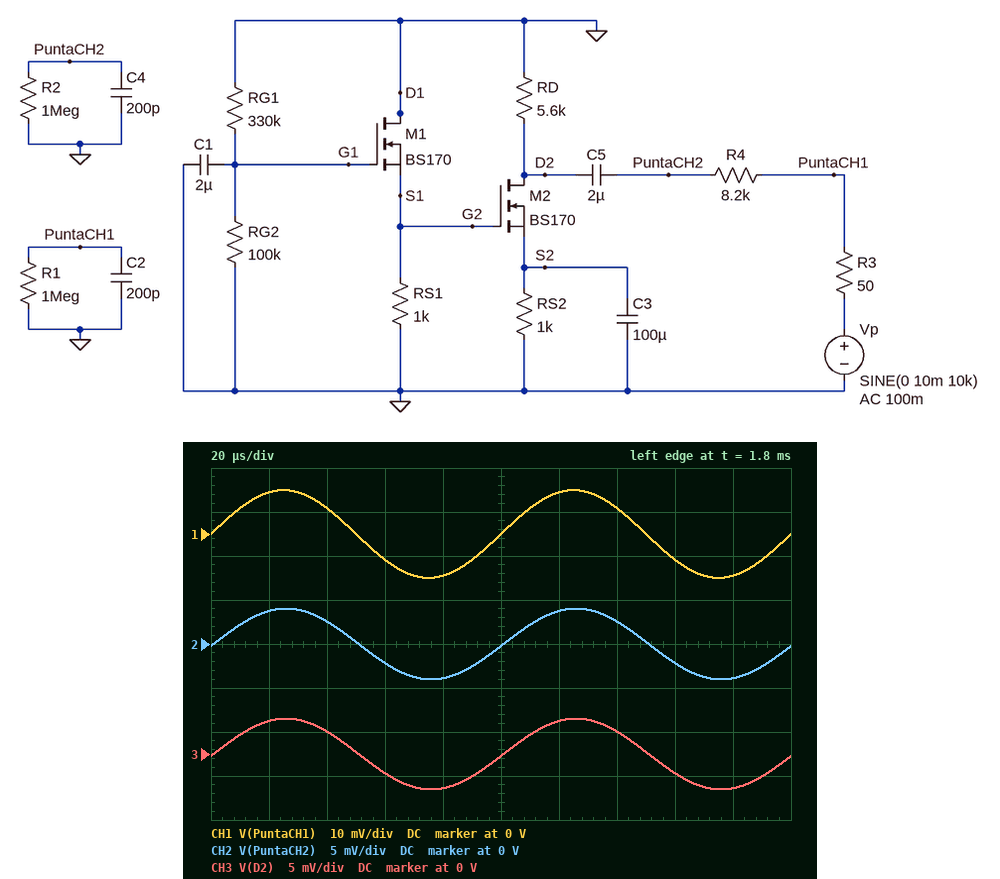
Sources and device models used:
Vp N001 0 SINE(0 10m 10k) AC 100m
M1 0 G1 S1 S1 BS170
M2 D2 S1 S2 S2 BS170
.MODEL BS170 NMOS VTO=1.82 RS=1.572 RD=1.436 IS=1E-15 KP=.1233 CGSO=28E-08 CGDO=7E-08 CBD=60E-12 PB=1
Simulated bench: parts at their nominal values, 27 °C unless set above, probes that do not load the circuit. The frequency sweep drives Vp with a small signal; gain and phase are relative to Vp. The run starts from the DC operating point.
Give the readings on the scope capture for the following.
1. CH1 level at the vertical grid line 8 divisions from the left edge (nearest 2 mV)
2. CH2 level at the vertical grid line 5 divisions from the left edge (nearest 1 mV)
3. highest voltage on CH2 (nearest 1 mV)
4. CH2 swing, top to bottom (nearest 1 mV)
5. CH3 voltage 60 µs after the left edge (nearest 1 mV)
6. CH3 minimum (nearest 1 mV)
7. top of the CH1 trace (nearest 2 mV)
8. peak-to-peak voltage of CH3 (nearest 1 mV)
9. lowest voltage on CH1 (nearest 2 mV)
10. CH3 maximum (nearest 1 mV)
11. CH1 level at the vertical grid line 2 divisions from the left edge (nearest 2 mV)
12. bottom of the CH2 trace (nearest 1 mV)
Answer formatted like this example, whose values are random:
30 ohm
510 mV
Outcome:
-6 mV
0 V
4 mV
8 mV
-2 mV
-4 mV
10 mV
8 mV
-10 mV
4 mV
6 mV
-4 mV
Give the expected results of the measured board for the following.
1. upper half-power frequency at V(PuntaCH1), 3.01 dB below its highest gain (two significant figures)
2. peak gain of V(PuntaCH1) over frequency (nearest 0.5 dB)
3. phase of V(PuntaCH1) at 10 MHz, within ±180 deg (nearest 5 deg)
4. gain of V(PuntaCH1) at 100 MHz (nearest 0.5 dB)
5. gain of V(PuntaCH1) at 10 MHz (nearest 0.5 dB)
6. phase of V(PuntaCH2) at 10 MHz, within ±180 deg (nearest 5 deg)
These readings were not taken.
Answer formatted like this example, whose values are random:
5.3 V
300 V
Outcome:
16 MHz
0 dB
-30 deg
-16.0 dB
-1.5 dB
-120 deg
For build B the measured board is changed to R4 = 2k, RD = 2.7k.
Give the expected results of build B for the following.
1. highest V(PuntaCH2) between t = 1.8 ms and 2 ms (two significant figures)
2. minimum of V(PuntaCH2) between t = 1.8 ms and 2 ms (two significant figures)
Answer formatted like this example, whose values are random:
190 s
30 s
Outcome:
5.7 mV
-5.7 mV
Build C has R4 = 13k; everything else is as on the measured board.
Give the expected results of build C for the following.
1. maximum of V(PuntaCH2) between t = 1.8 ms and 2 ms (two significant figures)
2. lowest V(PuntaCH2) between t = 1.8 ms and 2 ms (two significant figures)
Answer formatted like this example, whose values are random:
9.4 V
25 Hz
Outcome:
3.0 mV
-3.0 mV
